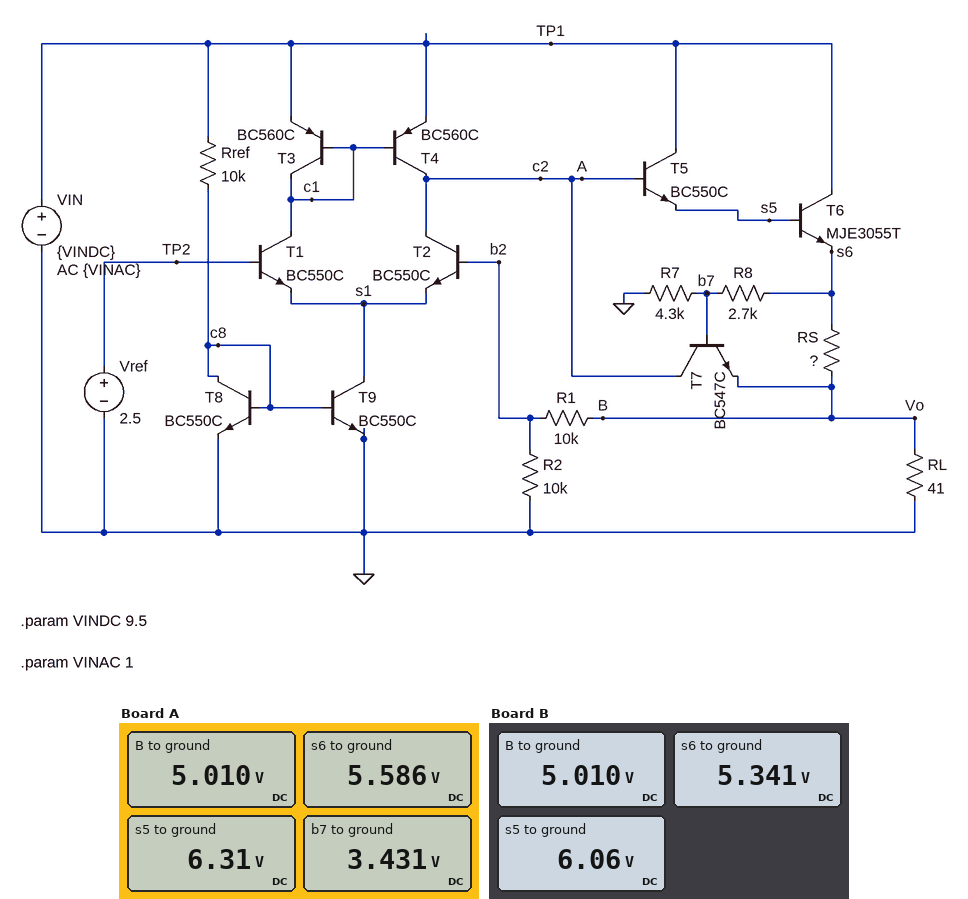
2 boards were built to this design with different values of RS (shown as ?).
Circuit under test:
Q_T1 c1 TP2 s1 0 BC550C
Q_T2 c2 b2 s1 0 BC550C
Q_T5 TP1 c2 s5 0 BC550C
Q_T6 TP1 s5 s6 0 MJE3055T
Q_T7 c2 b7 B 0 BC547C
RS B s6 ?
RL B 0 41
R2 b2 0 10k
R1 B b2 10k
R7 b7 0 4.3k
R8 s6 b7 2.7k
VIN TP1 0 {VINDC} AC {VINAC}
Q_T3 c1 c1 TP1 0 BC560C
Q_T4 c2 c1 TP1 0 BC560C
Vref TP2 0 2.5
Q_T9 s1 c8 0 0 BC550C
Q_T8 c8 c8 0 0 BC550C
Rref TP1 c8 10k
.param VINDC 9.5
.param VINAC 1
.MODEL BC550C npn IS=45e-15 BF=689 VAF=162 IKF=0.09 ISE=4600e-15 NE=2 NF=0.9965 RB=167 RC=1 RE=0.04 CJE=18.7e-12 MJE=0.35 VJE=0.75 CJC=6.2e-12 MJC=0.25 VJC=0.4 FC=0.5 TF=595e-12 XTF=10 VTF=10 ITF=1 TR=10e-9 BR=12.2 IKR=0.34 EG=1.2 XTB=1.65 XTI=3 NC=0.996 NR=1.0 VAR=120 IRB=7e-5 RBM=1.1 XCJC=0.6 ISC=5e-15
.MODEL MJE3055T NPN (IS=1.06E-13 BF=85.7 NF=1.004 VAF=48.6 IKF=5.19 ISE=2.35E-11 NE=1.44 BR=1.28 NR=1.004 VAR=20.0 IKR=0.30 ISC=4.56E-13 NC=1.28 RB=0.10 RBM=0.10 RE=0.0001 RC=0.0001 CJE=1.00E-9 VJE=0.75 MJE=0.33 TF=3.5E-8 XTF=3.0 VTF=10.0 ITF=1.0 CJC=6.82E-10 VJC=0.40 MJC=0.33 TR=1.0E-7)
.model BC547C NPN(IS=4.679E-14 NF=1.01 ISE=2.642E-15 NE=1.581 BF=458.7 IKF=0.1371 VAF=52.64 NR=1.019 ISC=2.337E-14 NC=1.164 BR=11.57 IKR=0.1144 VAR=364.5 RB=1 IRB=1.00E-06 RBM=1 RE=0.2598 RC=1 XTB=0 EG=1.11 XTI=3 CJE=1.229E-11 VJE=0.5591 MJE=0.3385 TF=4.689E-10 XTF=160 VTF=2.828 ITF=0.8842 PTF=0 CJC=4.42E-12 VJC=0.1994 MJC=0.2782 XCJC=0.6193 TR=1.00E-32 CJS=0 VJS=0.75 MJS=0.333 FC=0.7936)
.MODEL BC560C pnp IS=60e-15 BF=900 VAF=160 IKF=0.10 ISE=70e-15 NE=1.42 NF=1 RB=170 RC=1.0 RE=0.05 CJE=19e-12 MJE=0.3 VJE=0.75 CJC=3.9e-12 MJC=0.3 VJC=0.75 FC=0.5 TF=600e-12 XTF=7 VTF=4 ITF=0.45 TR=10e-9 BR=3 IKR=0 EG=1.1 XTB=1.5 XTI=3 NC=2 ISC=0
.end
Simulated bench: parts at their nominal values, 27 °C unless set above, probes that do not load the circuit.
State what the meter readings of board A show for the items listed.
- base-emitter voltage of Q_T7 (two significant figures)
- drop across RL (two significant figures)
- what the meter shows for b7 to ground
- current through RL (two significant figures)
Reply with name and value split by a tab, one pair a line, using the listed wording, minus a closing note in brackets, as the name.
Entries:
base-emitter voltage of Q_T7	-1.6 V
drop across RL	5.0 V
what the meter shows for b7 to ground	3.431 V
current through RL	120 mA
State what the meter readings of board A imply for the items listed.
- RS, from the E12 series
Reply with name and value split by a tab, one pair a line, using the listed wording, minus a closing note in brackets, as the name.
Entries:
RS, from the E12 series	4.7 Ω
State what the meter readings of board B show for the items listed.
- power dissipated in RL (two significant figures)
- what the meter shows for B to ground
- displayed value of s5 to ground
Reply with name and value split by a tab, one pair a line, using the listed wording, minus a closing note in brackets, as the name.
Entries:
power dissipated in RL	610 mW
what the meter shows for B to ground	5.010 V
displayed value of s5 to ground	6.06 V
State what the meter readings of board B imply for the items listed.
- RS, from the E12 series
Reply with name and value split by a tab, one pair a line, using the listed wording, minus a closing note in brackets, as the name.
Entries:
RS, from the E12 series	2.7 Ω
